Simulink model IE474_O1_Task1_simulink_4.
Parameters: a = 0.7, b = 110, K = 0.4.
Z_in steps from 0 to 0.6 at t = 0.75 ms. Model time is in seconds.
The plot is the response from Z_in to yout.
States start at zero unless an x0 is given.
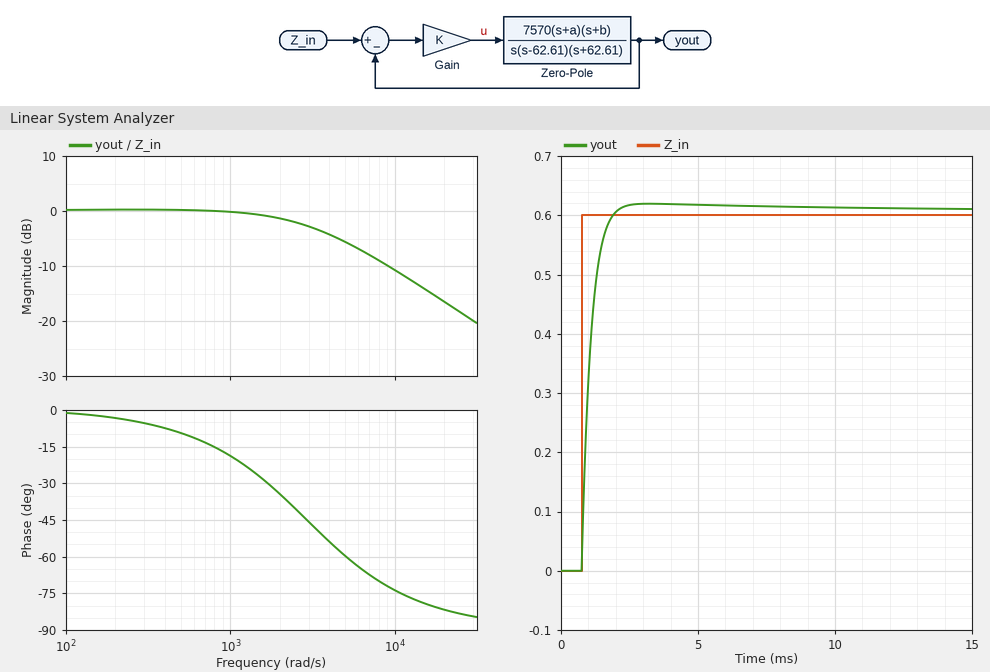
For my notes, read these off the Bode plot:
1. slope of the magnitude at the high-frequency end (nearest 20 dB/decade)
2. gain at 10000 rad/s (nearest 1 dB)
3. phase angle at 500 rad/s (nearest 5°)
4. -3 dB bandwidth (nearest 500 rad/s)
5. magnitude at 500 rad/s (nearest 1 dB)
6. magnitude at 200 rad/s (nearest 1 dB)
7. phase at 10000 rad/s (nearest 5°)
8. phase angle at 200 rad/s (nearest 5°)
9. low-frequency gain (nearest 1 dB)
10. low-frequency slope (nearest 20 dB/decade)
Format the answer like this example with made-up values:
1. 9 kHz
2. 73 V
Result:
1. -20 dB/decade
2. -11 dB
3. -10°
4. 3000 rad/s
5. 0 dB
6. 0 dB
7. -75°
8. -5°
9. 0 dB
10. 0 dB/decade
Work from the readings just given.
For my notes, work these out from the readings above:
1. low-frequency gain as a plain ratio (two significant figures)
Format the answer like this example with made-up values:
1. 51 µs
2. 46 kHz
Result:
1. 1.0
